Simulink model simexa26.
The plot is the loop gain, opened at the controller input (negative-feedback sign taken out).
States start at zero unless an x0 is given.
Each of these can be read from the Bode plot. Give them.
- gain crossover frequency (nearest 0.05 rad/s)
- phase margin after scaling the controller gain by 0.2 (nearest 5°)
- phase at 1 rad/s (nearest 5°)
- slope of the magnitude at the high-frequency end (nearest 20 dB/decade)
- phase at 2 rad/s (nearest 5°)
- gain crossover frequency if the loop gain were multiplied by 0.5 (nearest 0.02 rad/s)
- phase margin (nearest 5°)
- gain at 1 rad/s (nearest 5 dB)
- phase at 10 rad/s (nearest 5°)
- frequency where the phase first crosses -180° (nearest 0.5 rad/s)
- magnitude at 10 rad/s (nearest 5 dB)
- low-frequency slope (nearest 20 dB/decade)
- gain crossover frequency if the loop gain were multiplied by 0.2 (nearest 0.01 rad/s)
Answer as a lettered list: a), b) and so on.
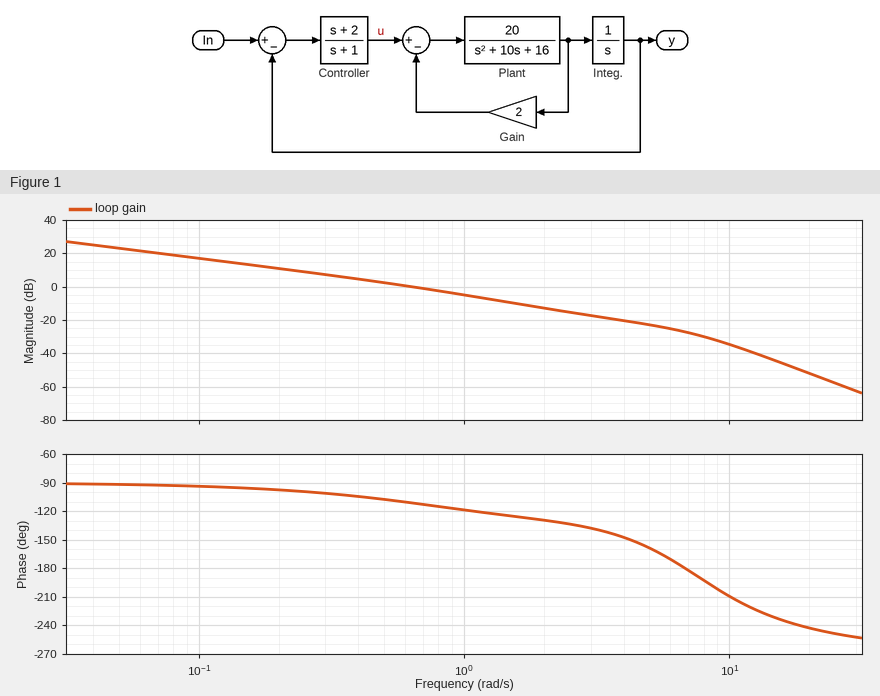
a) 0.65 rad/s
b) 85°
c) -120°
d) -60 dB/decade
e) -130°
f) 0.34 rad/s
g) 70°
h) -5 dB
i) -210°
j) 7.0 rad/s
k) -35 dB
l) -20 dB/decade
m) 0.14 rad/s
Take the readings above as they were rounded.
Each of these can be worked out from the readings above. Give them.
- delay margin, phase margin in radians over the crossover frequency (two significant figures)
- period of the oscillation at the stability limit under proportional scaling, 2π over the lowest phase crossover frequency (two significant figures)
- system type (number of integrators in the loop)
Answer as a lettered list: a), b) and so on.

a) 1.9 s
b) 0.90 s
c) 1
